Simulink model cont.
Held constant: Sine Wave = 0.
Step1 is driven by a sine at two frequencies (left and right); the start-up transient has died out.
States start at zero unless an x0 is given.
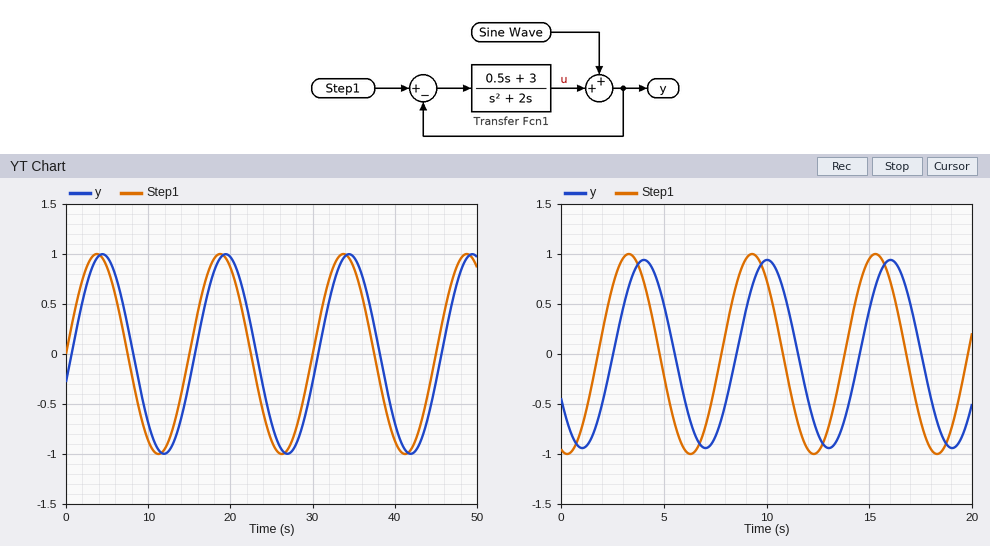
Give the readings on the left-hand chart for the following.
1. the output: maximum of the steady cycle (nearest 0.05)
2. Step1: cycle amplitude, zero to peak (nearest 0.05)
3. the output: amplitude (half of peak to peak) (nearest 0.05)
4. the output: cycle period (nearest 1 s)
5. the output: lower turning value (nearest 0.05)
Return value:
1.00
1.00
1.00
15 s
-1.00
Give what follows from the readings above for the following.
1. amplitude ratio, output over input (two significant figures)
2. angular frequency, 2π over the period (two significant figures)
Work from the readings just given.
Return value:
1.0
0.42 rad/s
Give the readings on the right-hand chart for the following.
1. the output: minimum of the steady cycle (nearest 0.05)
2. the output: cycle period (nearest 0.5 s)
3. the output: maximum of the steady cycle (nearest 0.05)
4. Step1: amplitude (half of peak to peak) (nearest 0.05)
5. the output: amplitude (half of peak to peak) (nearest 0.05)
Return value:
-0.95
6.0 s
0.95
1.00
0.95
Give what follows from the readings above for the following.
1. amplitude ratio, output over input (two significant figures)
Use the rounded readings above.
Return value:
0.95
